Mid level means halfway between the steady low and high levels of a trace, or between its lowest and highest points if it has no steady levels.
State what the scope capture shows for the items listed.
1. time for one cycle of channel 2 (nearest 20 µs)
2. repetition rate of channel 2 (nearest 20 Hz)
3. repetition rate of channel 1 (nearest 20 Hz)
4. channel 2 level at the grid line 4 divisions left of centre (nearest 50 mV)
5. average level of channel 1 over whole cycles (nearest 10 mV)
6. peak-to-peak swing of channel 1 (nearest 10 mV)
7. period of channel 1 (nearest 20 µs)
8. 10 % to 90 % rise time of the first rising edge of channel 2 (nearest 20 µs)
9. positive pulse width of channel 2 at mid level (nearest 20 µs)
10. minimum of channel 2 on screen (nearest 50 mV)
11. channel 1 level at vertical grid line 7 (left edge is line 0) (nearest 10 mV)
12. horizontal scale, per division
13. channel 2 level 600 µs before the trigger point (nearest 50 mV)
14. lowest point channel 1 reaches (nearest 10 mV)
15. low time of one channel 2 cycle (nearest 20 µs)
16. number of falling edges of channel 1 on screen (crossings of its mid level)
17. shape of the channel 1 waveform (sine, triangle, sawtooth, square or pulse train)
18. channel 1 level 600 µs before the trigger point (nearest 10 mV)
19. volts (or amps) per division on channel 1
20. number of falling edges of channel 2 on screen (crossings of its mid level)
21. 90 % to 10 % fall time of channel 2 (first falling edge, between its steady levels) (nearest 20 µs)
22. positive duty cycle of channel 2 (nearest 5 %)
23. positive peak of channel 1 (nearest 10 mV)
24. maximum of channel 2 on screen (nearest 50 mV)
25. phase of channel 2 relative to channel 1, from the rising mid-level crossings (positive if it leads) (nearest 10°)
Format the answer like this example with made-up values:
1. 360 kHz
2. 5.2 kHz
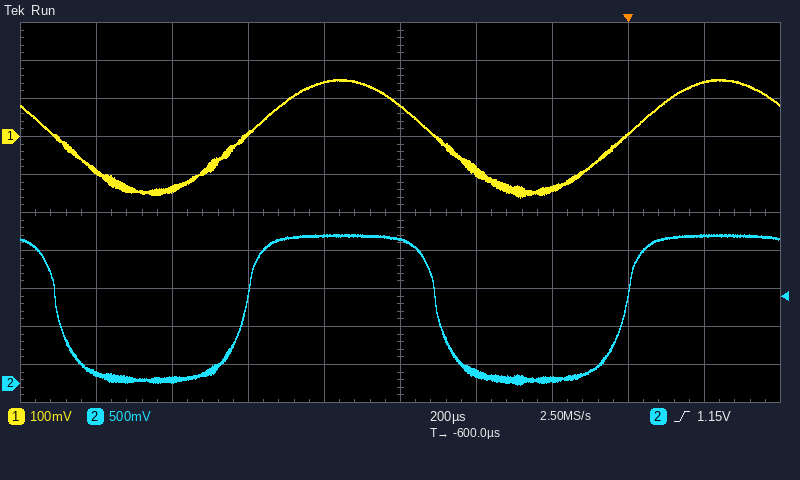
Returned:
1. 1.00 ms
2. 1.00 kHz
3. 1.00 kHz
4. 150 mV
5. 0 mV
6. 310 mV
7. 1.00 ms
8. 120 µs
9. 500 µs
10. 0 mV
11. -140 mV
12. 200 µs
13. 1.90 V
14. -160 mV
15. 500 µs
16. 2
17. sine
18. 80 mV
19. 100 mV
20. 2
21. 120 µs
22. 50 %
23. 150 mV
24. 1.95 V
25. 0°
